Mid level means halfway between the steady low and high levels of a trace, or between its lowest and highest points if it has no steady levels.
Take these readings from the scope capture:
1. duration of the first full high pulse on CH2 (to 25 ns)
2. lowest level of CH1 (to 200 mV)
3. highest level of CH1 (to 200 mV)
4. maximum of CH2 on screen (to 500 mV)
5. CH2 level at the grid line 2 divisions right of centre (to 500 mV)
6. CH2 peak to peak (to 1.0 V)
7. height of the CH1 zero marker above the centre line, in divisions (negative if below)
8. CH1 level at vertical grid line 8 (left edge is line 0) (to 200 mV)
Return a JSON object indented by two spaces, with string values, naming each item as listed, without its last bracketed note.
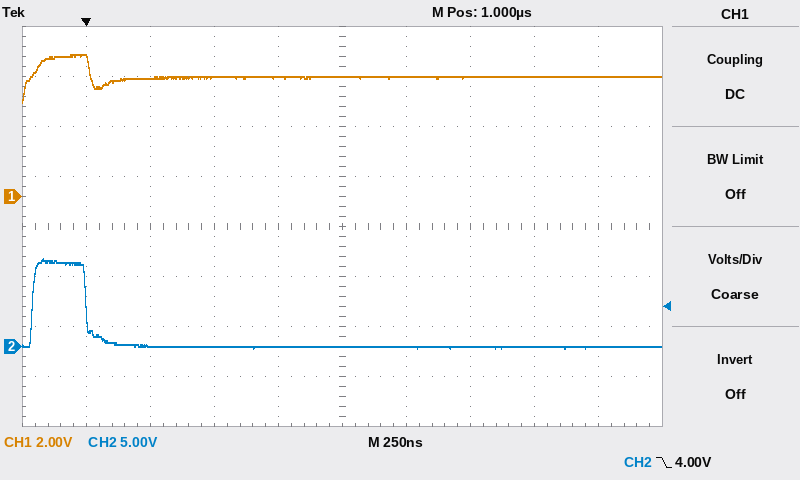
{
  "duration of the first full high pulse on CH2": "200 ns",
  "lowest level of CH1": "3.8 V",
  "highest level of CH1": "5.6 V",
  "maximum of CH2 on screen": "9.0 V",
  "CH2 level at the grid line 2 divisions right of centre": "0.0 V",
  "CH2 peak to peak": "9.0 V",
  "height of the CH1 zero marker above the centre line, in divisions": "+0.6 div",
  "CH1 level at vertical grid line 8 (left edge is line 0)": "4.8 V"
}
